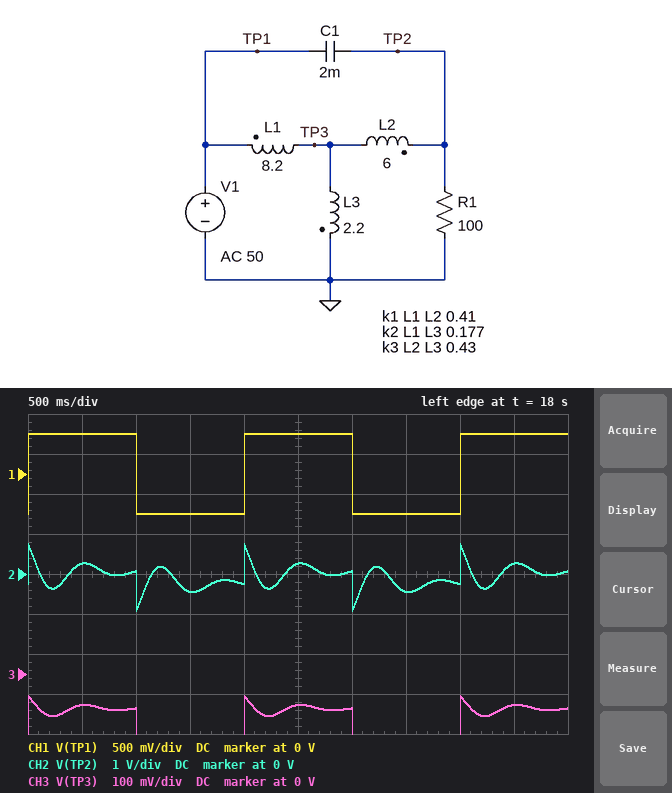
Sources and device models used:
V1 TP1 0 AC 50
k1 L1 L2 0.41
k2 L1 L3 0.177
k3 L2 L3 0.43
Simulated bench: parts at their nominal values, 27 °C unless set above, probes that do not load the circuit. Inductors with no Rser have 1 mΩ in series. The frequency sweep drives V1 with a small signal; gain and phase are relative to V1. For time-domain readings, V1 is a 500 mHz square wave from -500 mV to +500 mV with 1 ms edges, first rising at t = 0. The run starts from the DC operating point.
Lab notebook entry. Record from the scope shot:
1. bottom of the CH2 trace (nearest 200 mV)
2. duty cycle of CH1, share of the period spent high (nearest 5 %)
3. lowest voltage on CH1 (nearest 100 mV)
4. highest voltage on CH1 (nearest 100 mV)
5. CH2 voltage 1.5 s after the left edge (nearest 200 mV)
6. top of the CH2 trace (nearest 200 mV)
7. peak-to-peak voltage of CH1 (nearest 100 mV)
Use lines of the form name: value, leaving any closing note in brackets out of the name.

bottom of the CH2 trace: -1.0 V
duty cycle of CH1, share of the period spent high: 50 %
lowest voltage on CH1: -500 mV
highest voltage on CH1: 500 mV
CH2 voltage 1.5 s after the left edge: -400 mV
top of the CH2 trace: 800 mV
peak-to-peak voltage of CH1: 1.0 V
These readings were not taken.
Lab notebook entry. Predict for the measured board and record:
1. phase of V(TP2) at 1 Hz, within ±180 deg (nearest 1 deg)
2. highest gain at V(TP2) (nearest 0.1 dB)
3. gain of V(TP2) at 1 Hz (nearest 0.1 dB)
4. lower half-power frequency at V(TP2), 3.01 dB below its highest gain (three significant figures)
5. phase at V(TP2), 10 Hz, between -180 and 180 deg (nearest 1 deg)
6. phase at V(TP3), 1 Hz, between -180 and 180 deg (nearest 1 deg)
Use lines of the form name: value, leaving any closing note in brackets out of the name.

phase of V(TP2) at 1 Hz, within ±180 deg: 158 deg
highest gain at V(TP2): 4.3 dB
gain of V(TP2) at 1 Hz: -30.0 dB
lower half-power frequency at V(TP2), 3.01 dB below its highest gain: 1.58 Hz
phase at V(TP2), 10 Hz, between -180 and 180 deg: 5 deg
phase at V(TP3), 1 Hz, between -180 and 180 deg: 0 deg
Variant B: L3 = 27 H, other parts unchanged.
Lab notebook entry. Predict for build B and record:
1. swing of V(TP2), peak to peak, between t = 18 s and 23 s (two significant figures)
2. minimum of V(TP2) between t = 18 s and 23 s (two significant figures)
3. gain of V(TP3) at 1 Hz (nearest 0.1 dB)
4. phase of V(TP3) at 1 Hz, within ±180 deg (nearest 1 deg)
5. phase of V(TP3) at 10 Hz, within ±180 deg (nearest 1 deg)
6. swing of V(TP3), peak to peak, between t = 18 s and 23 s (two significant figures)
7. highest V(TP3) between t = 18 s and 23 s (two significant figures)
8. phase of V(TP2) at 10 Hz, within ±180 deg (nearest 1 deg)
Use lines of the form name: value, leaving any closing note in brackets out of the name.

swing of V(TP2), peak to peak, between t = 18 s and 23 s: 1.4 V
minimum of V(TP2) between t = 18 s and 23 s: -570 mV
gain of V(TP3) at 1 Hz: -5.0 dB
phase of V(TP3) at 1 Hz, within ±180 deg: -14 deg
phase of V(TP3) at 10 Hz, within ±180 deg: 3 deg
swing of V(TP3), peak to peak, between t = 18 s and 23 s: 1.2 V
highest V(TP3) between t = 18 s and 23 s: 760 mV
phase of V(TP2) at 10 Hz, within ±180 deg: 5 deg
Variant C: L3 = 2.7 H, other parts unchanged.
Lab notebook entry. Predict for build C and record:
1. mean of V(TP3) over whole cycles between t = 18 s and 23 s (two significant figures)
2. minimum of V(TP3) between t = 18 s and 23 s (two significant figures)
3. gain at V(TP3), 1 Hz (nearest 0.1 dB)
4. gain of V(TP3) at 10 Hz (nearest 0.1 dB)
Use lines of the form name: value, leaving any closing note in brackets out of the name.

mean of V(TP3) over whole cycles between t = 18 s and 23 s: -150 mV
minimum of V(TP3) between t = 18 s and 23 s: -310 mV
gain at V(TP3), 1 Hz: -15.2 dB
gain of V(TP3) at 10 Hz: -11.7 dB
